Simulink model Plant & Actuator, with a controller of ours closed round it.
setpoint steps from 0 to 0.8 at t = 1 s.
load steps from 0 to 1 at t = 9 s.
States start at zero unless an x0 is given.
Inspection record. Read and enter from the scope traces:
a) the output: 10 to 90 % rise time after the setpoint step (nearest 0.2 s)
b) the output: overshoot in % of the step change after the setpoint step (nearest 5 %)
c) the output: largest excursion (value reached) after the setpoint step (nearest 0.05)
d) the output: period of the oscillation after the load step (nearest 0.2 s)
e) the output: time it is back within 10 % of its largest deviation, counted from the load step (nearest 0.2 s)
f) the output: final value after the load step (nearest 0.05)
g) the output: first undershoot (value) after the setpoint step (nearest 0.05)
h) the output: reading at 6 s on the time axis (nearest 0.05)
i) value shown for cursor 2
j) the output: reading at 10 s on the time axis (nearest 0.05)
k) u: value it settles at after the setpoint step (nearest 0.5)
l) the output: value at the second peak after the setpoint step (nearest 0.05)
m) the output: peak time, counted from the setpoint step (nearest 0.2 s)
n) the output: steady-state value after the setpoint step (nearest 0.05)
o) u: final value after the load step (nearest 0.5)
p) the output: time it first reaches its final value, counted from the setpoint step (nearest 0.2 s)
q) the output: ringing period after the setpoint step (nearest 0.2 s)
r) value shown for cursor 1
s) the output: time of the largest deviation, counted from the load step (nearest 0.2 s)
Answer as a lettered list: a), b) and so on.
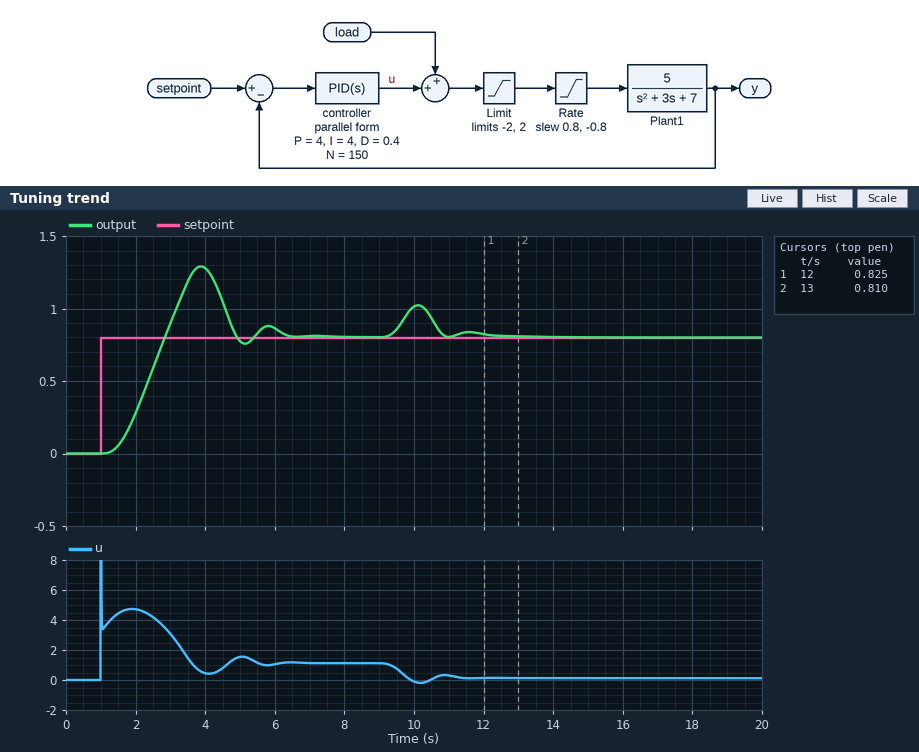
a) 1.2 s
b) 60 %
c) 1.30
d) 1.4 s
e) 3.0 s
f) 0.80
g) 0.75
h) 0.85
i) 0.810
j) 1.00
k) 1.0
l) 0.90
m) 2.8 s
n) 0.80
o) 0.0
p) 1.8 s
q) 2.0 s
r) 0.825
s) 1.2 s
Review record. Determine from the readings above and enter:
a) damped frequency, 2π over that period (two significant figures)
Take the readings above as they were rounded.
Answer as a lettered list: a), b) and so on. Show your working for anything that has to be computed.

a) 2π / 2 = 3.1 rad/s
